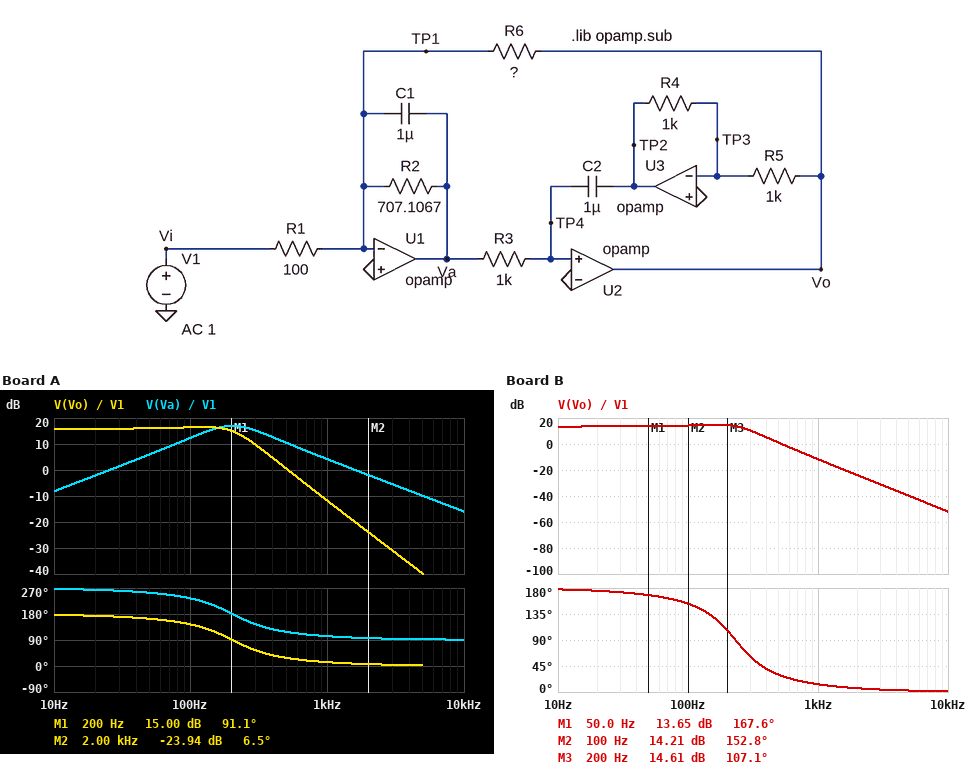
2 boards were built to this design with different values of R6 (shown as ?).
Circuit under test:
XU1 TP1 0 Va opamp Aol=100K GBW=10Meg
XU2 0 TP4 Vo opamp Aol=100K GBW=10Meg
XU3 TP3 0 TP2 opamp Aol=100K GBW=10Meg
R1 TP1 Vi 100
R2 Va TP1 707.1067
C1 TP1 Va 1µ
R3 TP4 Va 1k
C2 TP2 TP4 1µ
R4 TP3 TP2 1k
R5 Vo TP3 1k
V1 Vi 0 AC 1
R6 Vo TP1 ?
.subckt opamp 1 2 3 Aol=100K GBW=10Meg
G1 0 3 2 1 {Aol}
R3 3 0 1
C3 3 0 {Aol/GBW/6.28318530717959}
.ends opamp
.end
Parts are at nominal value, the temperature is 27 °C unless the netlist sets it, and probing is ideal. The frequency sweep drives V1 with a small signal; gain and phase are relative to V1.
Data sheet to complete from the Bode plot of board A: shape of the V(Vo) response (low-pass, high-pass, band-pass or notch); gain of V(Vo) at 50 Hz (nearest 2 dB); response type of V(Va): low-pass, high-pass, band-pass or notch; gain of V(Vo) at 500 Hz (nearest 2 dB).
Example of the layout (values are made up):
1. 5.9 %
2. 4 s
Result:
1. low-pass
2. 16 dB
3. band-pass
4. 0 dB
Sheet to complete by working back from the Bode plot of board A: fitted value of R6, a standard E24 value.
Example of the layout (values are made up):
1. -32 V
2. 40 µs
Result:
1. 620 Ω
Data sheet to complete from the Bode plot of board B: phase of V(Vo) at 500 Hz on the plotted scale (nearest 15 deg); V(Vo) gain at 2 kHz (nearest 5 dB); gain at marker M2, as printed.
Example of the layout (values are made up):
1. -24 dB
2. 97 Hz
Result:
1. 30 deg
2. -25 dB
3. 14.21 dB
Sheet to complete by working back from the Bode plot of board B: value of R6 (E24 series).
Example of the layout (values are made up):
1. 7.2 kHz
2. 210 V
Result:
1. 470 Ω
